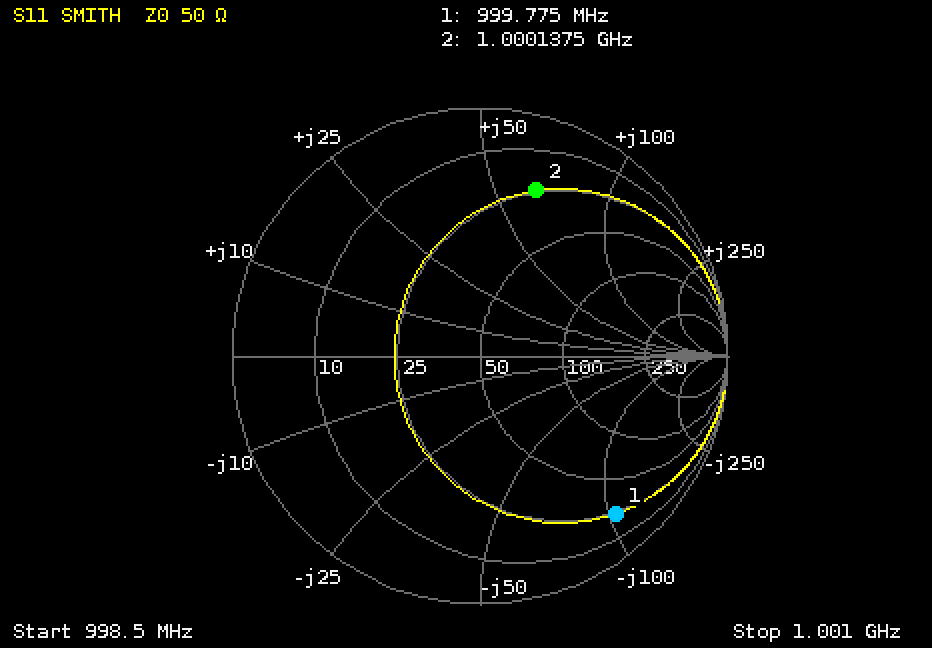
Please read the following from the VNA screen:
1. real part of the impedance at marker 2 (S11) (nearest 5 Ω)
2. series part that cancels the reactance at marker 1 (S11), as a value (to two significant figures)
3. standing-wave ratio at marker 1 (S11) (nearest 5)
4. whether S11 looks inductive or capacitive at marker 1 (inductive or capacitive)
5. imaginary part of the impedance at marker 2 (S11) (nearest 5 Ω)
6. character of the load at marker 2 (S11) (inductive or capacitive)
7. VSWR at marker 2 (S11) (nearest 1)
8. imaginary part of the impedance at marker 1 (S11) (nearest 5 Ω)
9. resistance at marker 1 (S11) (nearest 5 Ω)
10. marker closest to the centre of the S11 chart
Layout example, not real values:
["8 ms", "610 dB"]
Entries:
["25 Ω", "17 nH", "10", "capacitive", "+65 Ω", "inductive", "6", "-105 Ω", "25 Ω", "marker 2"]
